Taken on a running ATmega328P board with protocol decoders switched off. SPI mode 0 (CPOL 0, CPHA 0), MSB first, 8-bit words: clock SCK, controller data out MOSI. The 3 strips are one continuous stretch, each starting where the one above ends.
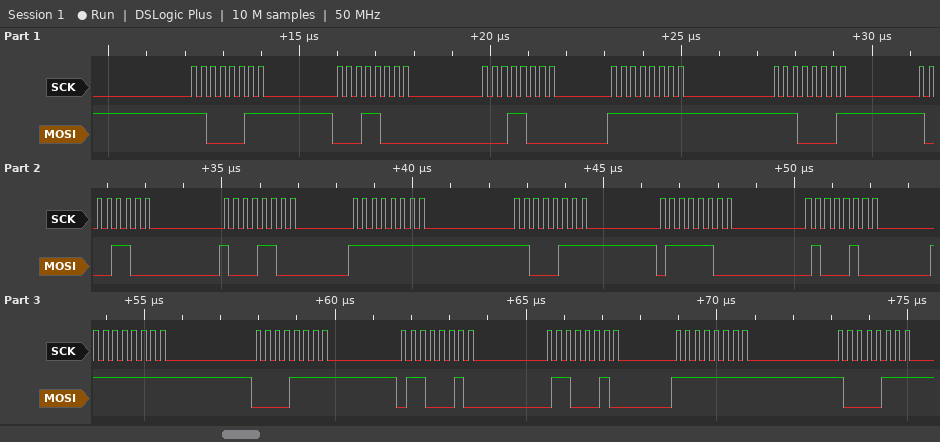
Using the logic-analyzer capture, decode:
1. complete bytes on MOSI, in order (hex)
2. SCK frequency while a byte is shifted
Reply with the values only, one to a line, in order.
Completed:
C3 18 18 FF E1 8C 8C FF C7 7C 44 FF 0F 62 62 FF 87
4 MHz
